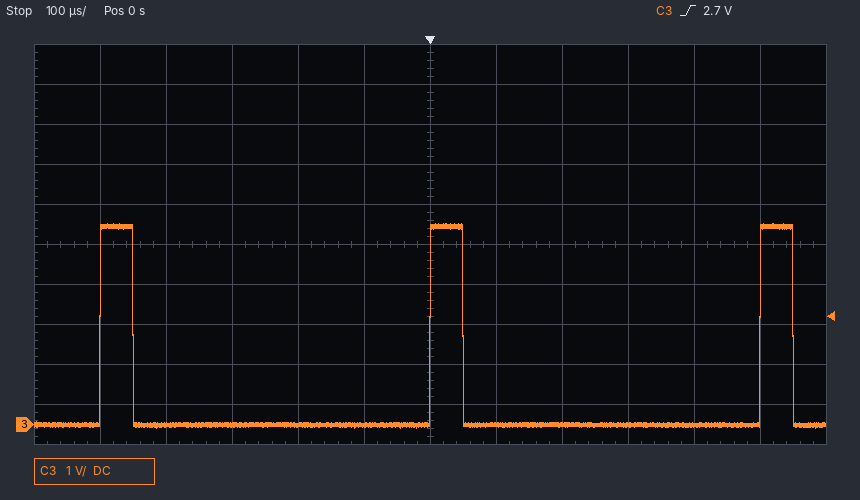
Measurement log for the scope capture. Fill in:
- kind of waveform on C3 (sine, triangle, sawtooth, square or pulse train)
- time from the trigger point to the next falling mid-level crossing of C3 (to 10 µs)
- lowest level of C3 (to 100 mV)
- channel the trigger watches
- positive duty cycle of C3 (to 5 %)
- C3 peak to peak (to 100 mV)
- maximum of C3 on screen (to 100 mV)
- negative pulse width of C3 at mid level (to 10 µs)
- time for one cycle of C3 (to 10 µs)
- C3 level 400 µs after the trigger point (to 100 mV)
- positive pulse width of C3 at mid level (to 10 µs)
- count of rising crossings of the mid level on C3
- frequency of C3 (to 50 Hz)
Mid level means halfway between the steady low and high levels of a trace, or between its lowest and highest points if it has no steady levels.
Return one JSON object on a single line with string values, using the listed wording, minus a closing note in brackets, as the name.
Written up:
{"kind of waveform on C3": "pulse train", "time from the trigger point to the next falling mid-level crossing of C3": "50 µs", "lowest level of C3": "-100 mV", "channel the trigger watches": "C3", "positive duty cycle of C3": "10 %", "C3 peak to peak": "5.1 V", "maximum of C3 on screen": "5.0 V", "negative pulse width of C3 at mid level": "450 µs", "time for one cycle of C3": "500 µs", "C3 level 400 µs after the trigger point": "0.0 V", "positive pulse width of C3 at mid level": "50 µs", "count of rising crossings of the mid level on C3": "3", "frequency of C3": "2.00 kHz"}
